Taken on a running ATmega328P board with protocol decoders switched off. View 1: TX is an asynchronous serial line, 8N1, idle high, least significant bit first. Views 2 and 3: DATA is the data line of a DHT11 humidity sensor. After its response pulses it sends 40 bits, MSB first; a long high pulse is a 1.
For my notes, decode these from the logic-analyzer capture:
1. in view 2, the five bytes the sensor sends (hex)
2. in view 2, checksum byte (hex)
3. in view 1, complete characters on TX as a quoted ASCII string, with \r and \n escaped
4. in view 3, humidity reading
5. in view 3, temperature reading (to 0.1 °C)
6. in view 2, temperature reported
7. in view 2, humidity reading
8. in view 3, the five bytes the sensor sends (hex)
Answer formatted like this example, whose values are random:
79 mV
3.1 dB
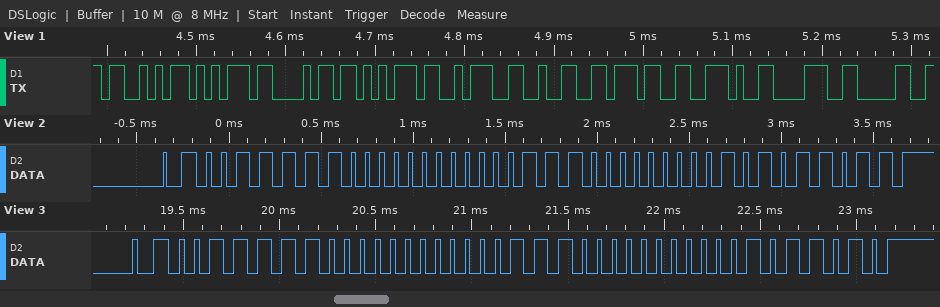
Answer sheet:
3E 00 1C 01 5B
0x5B
"Suhu:27.80"
62 %
28.0 °C
28.1 °C
62 %
3E 00 1C 00 5A
